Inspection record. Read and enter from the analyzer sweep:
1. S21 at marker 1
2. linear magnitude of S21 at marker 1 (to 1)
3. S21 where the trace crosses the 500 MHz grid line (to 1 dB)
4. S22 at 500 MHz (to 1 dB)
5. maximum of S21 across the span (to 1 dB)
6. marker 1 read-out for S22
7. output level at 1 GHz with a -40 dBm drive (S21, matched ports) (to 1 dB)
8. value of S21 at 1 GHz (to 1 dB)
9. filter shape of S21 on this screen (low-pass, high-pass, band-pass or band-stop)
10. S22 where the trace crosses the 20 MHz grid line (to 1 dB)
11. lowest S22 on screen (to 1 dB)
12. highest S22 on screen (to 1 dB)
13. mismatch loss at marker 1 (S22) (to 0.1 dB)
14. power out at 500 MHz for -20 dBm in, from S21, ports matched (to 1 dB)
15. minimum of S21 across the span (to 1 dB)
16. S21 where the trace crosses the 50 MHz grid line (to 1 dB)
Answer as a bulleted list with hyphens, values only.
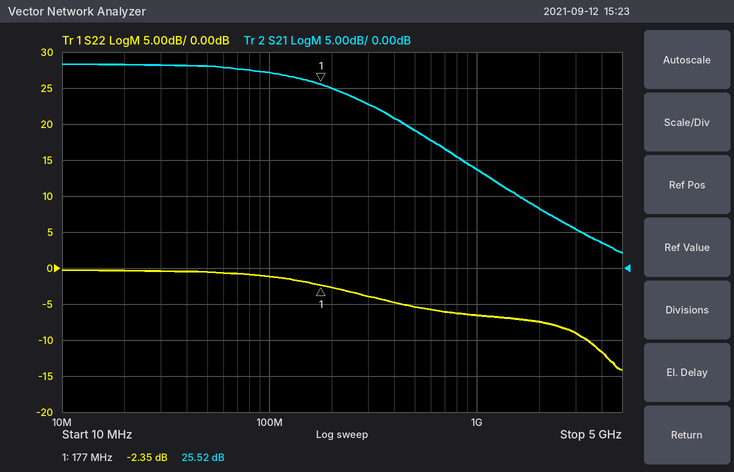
- 25.52 dB
- 19
- 19 dB
- -5 dB
- 28 dB
- -2.35 dB
- -26 dBm
- 14 dB
- low-pass
- 0 dB
- -14 dB
- 0 dB
- 3.8 dB
- -1 dBm
- 2 dB
- 28 dB
